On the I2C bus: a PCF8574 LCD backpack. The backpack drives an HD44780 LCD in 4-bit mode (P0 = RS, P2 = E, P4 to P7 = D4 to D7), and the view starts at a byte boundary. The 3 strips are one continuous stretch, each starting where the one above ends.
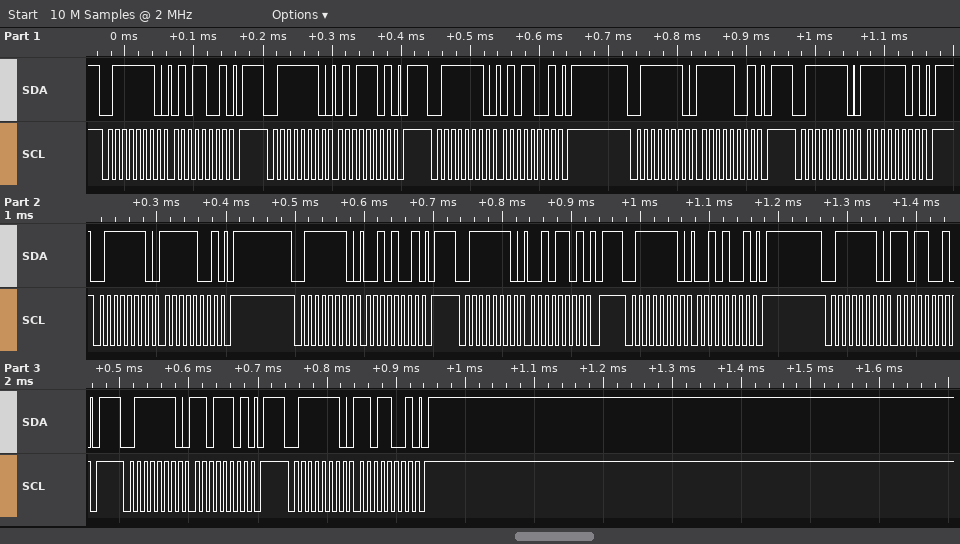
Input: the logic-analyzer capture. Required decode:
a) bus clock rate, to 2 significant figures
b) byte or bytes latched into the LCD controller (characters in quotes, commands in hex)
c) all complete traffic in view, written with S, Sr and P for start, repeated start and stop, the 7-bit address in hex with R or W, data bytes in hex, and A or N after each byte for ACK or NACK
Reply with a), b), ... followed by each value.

a) 100 kHz
b) '_' '-'
c) S 3FW A 59 A P S 3FW A 5D A P S 3FW A 59 A P S 3FW A F9 A P S 3FW A FD A P S 3FW A F9 A P S 3FW A 29 A P S 3FW A 2D A P S 3FW A 29 A P S 3FW A D9 A P S 3FW A DD A P S 3FW A D9 A P
